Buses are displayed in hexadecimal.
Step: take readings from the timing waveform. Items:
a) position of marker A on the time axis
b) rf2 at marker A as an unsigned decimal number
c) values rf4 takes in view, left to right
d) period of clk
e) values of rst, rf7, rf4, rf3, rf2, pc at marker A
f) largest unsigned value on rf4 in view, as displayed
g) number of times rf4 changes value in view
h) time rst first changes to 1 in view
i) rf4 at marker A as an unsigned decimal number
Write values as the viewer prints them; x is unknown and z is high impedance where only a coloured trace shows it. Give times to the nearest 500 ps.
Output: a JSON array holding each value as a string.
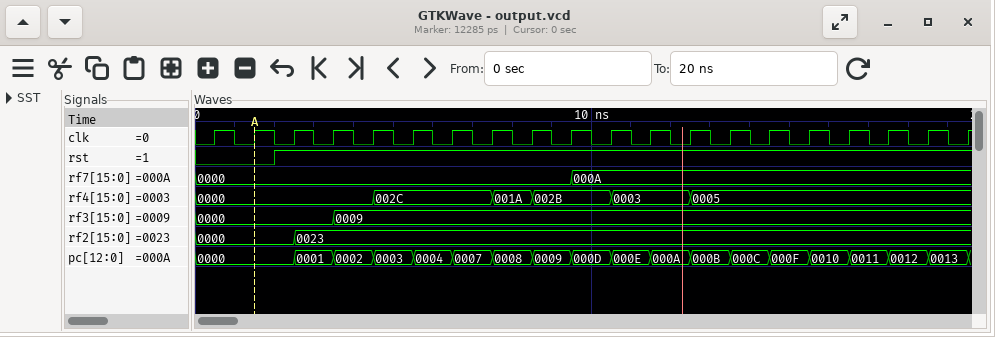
["1500 ps", "0", "0000, 002C, 001A, 002B, 0003, 0005", "1000 ps", "rst=0, rf7=0000, rf4=0000, rf3=0000, rf2=0000, pc=0000", "002C", "5", "2000 ps", "0"]
